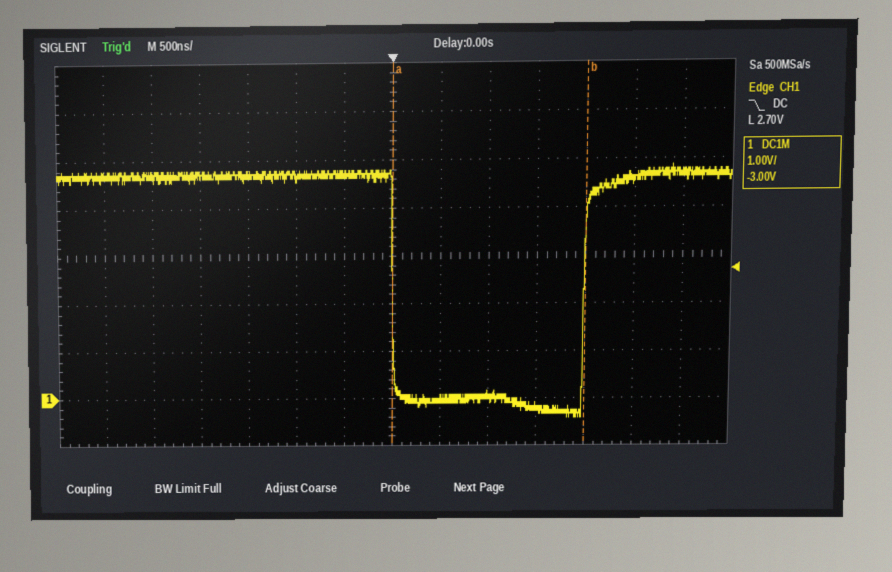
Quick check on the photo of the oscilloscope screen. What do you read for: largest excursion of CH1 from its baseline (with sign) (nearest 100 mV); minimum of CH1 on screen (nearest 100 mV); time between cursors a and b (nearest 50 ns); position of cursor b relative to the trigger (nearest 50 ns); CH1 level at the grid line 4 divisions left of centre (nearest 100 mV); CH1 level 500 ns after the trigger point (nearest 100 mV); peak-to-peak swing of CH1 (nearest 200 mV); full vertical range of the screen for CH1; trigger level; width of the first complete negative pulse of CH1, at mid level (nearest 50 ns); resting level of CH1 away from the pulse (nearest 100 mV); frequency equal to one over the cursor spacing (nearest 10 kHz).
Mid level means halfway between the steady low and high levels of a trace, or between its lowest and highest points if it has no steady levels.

-5.1 V
-400 mV
2.00 µs
+2.00 µs
4.7 V
0.0 V
5.2 V
8 V
2.70 V
2.00 µs
4.7 V
500 kHz
